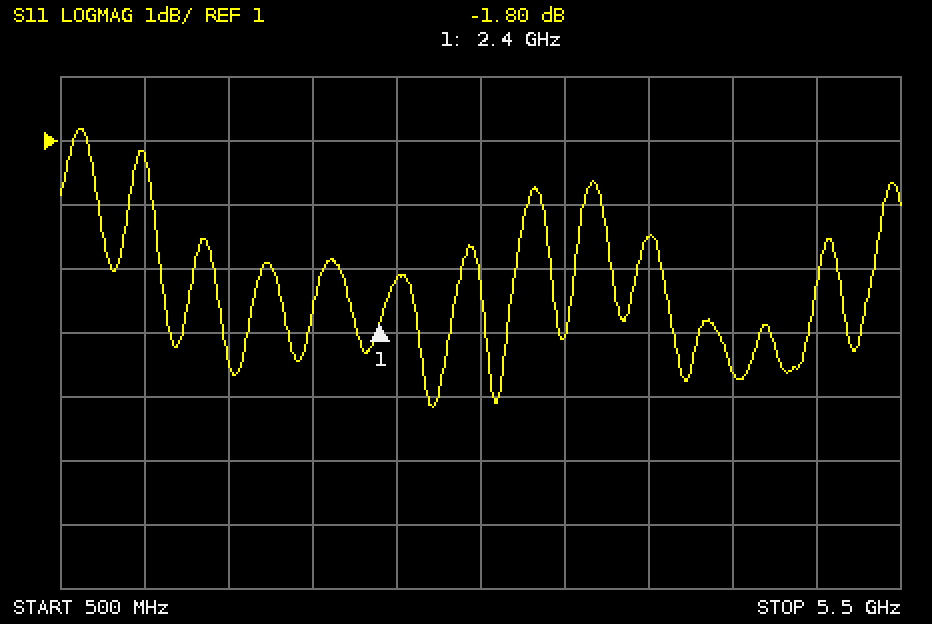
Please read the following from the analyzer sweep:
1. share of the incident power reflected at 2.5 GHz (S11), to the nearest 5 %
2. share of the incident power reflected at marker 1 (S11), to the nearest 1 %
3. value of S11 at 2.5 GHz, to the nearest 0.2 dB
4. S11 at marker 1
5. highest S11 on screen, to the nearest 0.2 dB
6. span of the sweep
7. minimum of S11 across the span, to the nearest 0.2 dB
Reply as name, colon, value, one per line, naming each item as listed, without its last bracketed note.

share of the incident power reflected at 2.5 GHz (S11), to the nearest 5 %: 75 %
share of the incident power reflected at marker 1 (S11), to the nearest 1 %: 66 %
value of S11 at 2.5 GHz, to the nearest 0.2 dB: -1.2 dB
S11 at marker 1: -1.80 dB
highest S11 on screen, to the nearest 0.2 dB: 1.2 dB
span of the sweep: 5 GHz
minimum of S11 across the span, to the nearest 0.2 dB: -3.2 dB
